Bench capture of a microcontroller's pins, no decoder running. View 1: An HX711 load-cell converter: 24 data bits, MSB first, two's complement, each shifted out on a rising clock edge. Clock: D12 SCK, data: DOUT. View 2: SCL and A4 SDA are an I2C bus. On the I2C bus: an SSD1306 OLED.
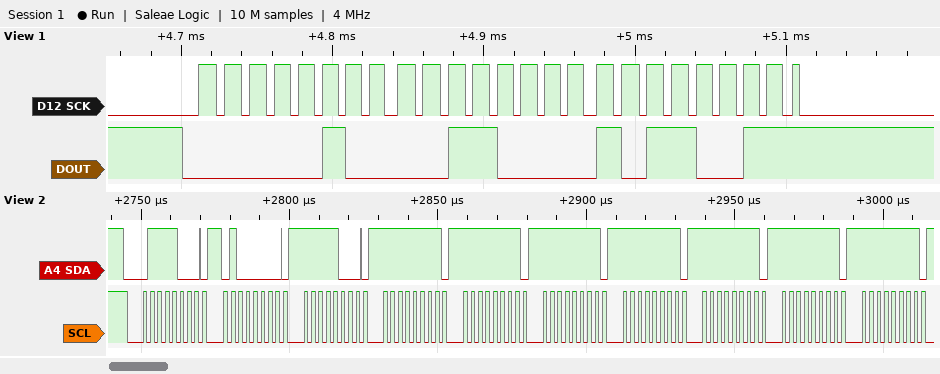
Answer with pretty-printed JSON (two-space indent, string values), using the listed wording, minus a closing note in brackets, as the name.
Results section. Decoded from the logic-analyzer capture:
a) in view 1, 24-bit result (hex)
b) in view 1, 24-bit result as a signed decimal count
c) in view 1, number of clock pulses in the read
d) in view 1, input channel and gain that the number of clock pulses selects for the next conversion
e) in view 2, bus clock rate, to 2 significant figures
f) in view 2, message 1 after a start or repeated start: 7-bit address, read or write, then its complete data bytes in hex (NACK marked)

{
  "in view 1, 24-bit result": "0x0430B3",
  "in view 1, 24-bit result as a signed decimal count": "274611",
  "in view 1, number of clock pulses in the read": "25",
  "in view 1, input channel and gain that the number of clock pulses selects for the next conversion": "channel A, gain 128",
  "in view 2, bus clock rate, to 2 significant figures": "400 kHz",
  "in view 2, message 1 after a start or repeated start: 7-bit address, read or write, then its complete data bytes in hex": "0x3C write: 40 F8 FF FF FF FF FF FF FF"
}
